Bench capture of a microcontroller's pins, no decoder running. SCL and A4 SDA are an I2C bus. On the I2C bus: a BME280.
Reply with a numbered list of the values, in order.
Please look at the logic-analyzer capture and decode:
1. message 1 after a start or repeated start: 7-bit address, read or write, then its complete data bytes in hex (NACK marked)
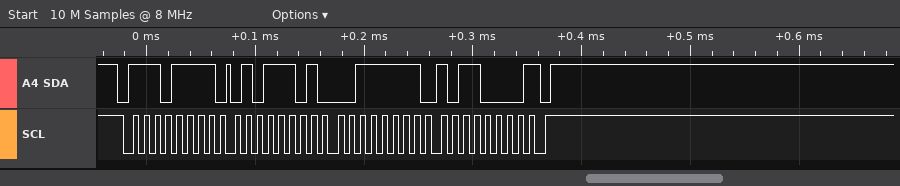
1. 0x77 read: 5D 3F B0 NACK
